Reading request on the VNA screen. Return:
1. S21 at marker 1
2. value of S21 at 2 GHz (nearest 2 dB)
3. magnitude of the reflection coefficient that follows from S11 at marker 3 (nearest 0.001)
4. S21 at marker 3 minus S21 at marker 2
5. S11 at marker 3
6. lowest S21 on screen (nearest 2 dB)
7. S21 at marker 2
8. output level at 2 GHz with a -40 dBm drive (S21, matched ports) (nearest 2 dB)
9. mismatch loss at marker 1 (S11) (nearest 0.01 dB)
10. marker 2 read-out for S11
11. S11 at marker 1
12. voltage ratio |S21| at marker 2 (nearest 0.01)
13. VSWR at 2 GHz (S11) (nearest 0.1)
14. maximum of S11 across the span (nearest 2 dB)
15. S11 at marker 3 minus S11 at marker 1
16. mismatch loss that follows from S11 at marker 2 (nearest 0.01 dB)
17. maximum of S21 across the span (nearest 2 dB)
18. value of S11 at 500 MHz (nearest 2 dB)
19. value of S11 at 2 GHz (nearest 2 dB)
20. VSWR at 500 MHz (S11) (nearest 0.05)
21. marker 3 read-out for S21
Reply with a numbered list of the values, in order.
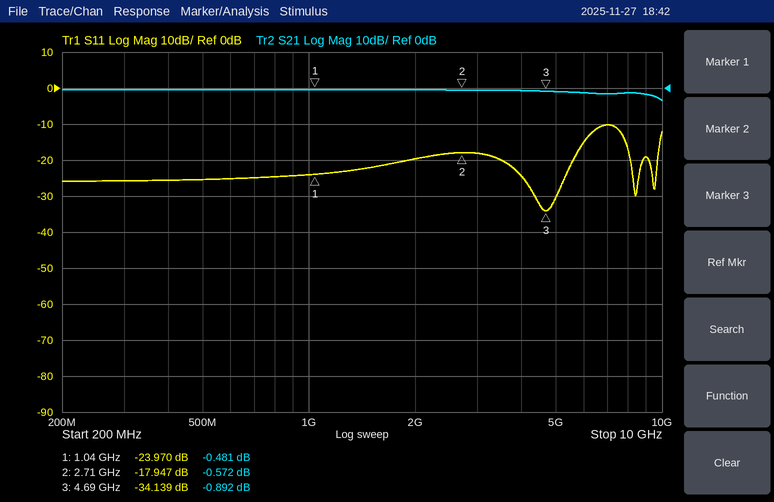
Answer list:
1. -0.481 dB
2. 0 dB
3. 0.020
4. -0.320 dB
5. -34.139 dB
6. -4 dB
7. -0.572 dB
8. -40 dBm
9. 0.02 dB
10. -17.947 dB
11. -23.970 dB
12. 0.94
13. 1.2
14. -10 dB
15. -10.169 dB
16. 0.07 dB
17. 0 dB
18. -26 dB
19. -20 dB
20. 1.10
21. -0.892 dB
